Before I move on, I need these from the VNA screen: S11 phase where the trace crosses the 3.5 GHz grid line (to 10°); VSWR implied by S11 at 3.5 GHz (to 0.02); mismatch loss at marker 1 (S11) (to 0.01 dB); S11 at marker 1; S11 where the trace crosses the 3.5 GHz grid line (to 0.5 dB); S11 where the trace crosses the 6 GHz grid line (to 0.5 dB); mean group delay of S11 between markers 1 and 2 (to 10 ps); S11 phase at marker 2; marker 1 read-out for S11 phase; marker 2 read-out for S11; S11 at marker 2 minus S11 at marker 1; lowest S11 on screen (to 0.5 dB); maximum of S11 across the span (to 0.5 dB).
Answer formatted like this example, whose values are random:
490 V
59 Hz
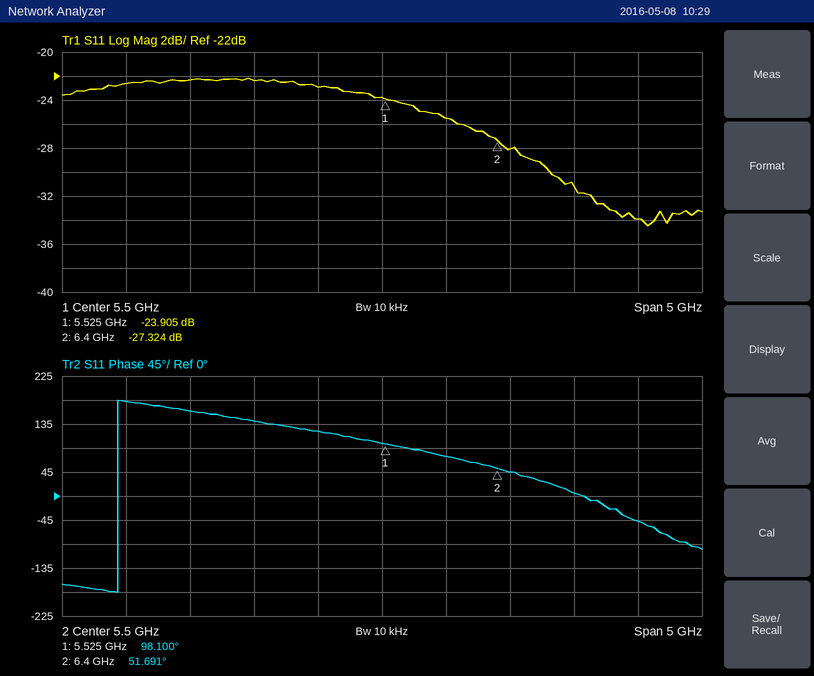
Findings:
180°
1.16
0.02 dB
-23.905 dB
-22.5 dB
-25.5 dB
150 ps
51.691°
98.100°
-27.324 dB
-3.419 dB
-34.5 dB
-22.0 dB
